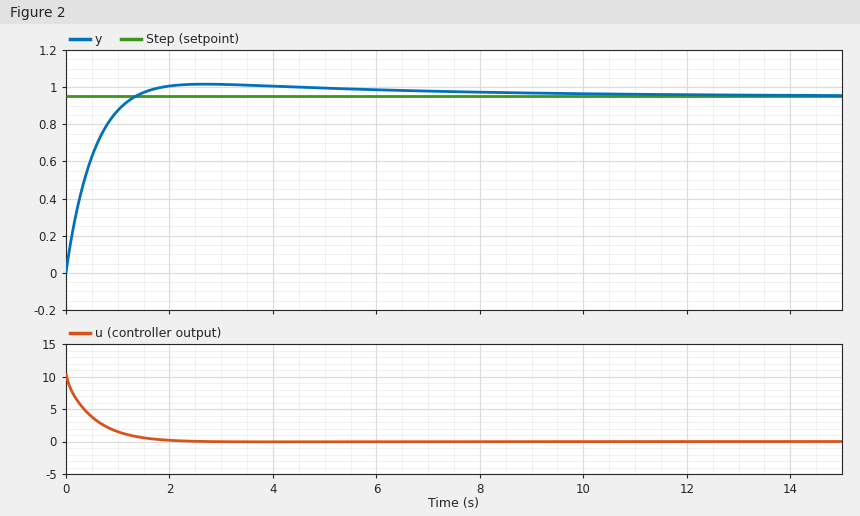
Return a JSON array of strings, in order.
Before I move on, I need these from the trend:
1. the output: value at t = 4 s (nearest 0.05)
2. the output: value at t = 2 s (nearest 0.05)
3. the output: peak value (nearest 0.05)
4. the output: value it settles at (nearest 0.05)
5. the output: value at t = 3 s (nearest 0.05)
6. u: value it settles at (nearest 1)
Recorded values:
["1.00", "1.00", "1.00", "0.95", "1.00", "0"]
